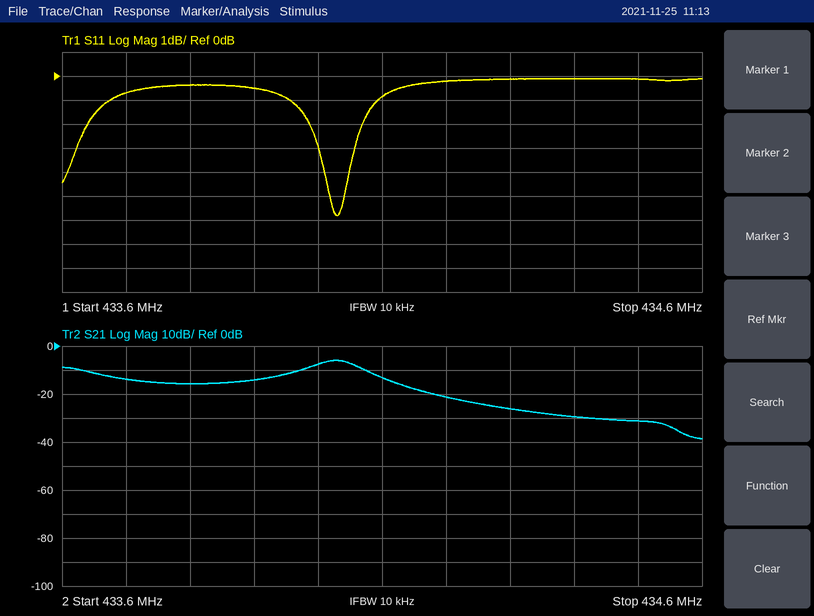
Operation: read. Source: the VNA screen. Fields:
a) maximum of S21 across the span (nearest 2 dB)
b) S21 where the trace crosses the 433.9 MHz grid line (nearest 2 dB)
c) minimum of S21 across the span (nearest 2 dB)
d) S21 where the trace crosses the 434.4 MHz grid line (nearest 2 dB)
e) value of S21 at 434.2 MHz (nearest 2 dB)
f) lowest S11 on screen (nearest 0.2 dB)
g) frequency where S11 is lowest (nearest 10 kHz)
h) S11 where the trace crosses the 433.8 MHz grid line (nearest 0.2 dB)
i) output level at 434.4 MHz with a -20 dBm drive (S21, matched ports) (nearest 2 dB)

-6 dB
-14 dB
-38 dB
-30 dB
-22 dB
-5.8 dB
434.03 MHz
-0.4 dB
-50 dBm
